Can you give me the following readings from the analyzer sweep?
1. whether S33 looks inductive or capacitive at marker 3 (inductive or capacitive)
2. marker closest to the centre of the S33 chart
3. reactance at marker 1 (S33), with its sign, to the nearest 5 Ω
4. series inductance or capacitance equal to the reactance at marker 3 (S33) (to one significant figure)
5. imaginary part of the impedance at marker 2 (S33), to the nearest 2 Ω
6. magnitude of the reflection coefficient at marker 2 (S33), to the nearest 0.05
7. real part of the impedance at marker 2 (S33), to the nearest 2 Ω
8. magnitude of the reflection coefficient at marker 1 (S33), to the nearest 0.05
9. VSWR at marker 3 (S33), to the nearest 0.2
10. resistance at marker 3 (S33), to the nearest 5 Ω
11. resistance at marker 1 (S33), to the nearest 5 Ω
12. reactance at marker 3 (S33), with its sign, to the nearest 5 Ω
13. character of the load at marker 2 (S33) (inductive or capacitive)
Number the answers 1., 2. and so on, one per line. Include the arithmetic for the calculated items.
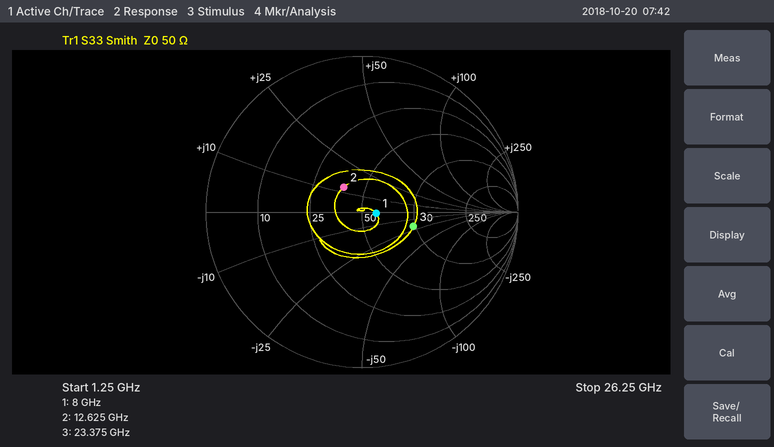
1. capacitive
2. marker 1
3. 0 Ω
4. C = 1/(2π × 23.375 GHz × 20 Ω) ≈ 340 fF, so 300 fF to one significant figure
5. +12 Ω
6. 0.20
7. 38 Ω
8. 0.10
9. 2.0
10. 95 Ω
11. 60 Ω
12. -20 Ω
13. inductive
